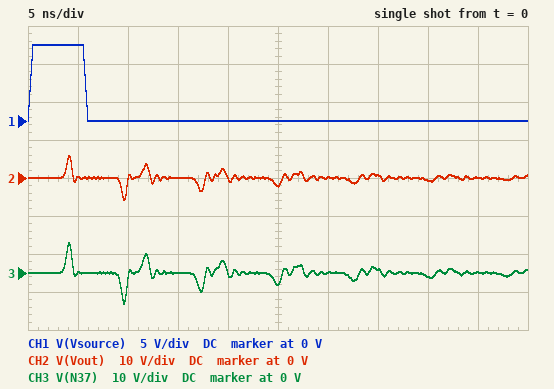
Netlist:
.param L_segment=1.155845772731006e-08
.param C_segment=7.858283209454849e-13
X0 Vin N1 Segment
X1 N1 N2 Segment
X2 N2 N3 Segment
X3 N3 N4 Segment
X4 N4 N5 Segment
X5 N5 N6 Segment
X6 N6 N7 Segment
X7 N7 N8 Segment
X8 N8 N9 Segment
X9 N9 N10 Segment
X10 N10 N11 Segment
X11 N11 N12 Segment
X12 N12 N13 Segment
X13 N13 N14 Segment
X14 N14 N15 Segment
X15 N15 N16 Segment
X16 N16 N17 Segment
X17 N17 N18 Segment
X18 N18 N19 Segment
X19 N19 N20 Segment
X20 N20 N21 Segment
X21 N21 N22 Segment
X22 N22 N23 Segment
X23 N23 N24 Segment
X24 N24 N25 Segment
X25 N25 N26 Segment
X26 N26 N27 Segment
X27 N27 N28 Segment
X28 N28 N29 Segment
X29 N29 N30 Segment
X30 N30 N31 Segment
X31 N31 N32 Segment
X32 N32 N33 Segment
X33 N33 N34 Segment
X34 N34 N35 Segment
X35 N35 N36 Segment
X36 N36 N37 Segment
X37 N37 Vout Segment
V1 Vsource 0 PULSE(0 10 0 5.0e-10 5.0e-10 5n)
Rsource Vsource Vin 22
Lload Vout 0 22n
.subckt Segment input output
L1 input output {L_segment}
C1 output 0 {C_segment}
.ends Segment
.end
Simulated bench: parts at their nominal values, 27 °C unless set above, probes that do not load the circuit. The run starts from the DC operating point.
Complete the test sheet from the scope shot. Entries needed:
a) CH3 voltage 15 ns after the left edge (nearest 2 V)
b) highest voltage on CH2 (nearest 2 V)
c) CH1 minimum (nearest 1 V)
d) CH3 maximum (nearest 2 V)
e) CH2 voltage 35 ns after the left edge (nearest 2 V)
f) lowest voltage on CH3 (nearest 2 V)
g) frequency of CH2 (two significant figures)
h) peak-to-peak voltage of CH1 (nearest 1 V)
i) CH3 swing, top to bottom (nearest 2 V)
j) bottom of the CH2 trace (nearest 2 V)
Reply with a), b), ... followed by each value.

a) 0 V
b) 6 V
c) 0 V
d) 8 V
e) 0 V
f) -8 V
g) 130 MHz
h) 10 V
i) 16 V
j) -6 V
